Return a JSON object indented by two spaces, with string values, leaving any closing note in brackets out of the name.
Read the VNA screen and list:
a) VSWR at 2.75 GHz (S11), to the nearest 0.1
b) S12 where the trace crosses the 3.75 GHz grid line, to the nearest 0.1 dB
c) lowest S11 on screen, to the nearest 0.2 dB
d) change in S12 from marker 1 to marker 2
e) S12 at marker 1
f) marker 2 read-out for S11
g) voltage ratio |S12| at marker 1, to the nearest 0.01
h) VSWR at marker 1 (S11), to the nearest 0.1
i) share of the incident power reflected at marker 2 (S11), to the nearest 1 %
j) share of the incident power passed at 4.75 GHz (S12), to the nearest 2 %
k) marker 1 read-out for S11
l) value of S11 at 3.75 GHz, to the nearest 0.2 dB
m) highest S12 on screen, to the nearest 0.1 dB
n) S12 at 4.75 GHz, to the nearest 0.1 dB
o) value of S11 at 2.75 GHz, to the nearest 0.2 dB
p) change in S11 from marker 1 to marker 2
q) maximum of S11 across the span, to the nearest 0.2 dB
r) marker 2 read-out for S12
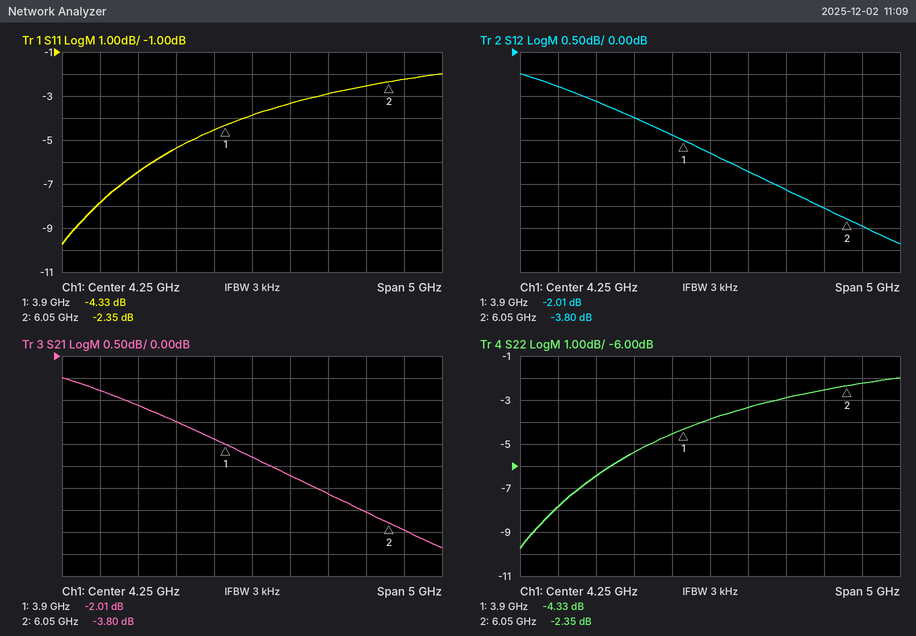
{
  "VSWR at 2.75 GHz (S11), to the nearest 0.1": "2.8",
  "S12 where the trace crosses the 3.75 GHz grid line, to the nearest 0.1 dB": "-1.9 dB",
  "lowest S11 on screen, to the nearest 0.2 dB": "-9.8 dB",
  "change in S12 from marker 1 to marker 2": "-1.79 dB",
  "S12 at marker 1": "-2.01 dB",
  "marker 2 read-out for S11": "-2.35 dB",
  "voltage ratio |S12| at marker 1, to the nearest 0.01": "0.79",
  "VSWR at marker 1 (S11), to the nearest 0.1": "4.1",
  "share of the incident power reflected at marker 2 (S11), to the nearest 1 %": "58 %",
  "share of the incident power passed at 4.75 GHz (S12), to the nearest 2 %": "54 %",
  "marker 1 read-out for S11": "-4.33 dB",
  "value of S11 at 3.75 GHz, to the nearest 0.2 dB": "-4.6 dB",
  "highest S12 on screen, to the nearest 0.1 dB": "-0.5 dB",
  "S12 at 4.75 GHz, to the nearest 0.1 dB": "-2.7 dB",
  "value of S11 at 2.75 GHz, to the nearest 0.2 dB": "-6.4 dB",
  "change in S11 from marker 1 to marker 2": "1.98 dB",
  "maximum of S11 across the span, to the nearest 0.2 dB": "-2.0 dB",
  "marker 2 read-out for S12": "-3.80 dB"
}
